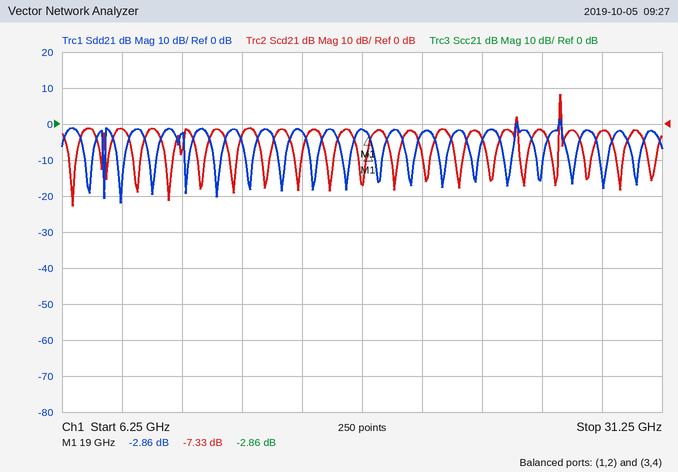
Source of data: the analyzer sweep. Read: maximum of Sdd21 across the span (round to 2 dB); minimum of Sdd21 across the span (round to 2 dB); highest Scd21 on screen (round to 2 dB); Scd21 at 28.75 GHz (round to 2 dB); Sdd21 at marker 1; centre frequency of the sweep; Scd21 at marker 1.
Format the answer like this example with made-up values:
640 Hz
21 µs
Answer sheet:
2 dB
-22 dB
8 dB
-2 dB
-2.86 dB
18.75 GHz
-7.33 dB
